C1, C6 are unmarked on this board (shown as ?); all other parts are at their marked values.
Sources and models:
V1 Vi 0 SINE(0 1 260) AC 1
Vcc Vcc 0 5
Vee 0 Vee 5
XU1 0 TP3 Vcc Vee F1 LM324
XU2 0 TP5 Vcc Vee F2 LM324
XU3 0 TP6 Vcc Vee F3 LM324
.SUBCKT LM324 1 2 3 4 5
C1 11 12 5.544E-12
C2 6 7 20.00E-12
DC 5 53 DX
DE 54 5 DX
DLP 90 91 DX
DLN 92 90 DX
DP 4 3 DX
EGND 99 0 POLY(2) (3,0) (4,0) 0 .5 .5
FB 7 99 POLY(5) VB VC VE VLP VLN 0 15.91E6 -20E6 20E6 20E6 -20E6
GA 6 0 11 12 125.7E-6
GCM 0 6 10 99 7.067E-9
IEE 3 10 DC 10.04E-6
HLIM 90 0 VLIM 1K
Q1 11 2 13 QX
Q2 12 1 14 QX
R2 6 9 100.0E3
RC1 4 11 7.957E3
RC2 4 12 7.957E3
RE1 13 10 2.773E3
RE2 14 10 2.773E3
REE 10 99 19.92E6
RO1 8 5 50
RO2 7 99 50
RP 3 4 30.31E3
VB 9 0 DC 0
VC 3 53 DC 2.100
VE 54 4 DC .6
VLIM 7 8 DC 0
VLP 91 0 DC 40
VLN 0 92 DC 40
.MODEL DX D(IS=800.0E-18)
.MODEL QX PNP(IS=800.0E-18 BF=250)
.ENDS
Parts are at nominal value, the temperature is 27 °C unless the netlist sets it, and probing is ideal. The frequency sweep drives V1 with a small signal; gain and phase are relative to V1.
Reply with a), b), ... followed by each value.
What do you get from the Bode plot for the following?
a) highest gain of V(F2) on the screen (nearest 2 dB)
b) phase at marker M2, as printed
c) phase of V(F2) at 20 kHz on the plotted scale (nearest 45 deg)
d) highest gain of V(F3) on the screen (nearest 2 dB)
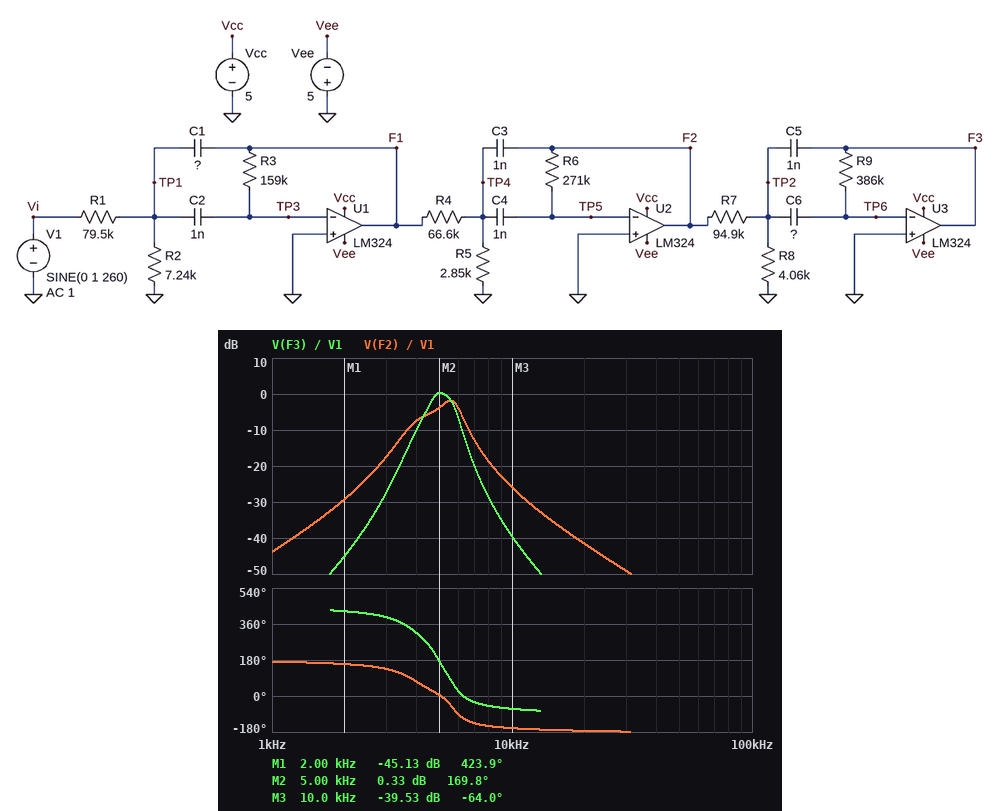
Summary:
a) -2 dB
b) 169.8 deg
c) -180 deg
d) 0 dB
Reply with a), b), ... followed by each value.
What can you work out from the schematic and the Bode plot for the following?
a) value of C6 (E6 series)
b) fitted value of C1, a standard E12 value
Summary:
a) 680 pF
b) 1.5 nF
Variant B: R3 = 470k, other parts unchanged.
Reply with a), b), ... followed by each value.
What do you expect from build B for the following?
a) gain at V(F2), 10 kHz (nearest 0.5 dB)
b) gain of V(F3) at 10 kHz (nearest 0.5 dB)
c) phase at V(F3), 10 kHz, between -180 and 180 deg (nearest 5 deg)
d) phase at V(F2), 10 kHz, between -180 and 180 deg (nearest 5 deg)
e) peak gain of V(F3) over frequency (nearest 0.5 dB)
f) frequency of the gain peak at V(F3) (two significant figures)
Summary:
a) -27.0 dB
b) -40.5 dB
c) -70 deg
d) -170 deg
e) -3.5 dB
f) 5.1 kHz
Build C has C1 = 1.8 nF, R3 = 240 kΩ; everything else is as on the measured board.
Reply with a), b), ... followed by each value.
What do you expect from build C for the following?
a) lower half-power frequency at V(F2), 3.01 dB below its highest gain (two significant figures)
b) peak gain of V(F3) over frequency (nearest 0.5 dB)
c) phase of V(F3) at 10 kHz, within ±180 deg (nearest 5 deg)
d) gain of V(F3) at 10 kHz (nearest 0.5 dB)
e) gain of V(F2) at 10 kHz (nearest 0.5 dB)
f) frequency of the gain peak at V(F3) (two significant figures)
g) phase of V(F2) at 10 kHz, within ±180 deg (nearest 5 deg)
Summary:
a) 4.9 kHz
b) -4.0 dB
c) -70 deg
d) -41.5 dB
e) -28.0 dB
f) 5.1 kHz
g) -165 deg
